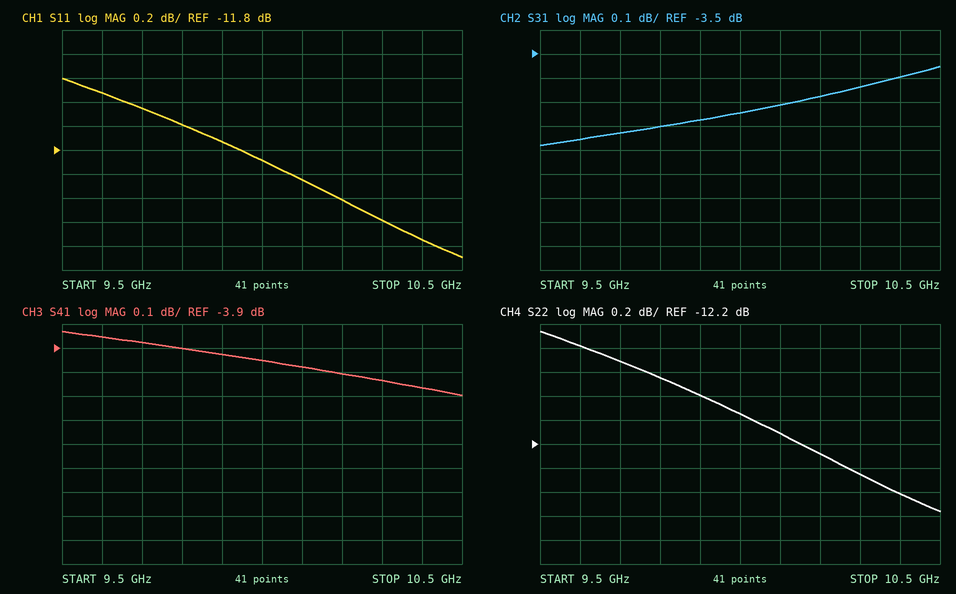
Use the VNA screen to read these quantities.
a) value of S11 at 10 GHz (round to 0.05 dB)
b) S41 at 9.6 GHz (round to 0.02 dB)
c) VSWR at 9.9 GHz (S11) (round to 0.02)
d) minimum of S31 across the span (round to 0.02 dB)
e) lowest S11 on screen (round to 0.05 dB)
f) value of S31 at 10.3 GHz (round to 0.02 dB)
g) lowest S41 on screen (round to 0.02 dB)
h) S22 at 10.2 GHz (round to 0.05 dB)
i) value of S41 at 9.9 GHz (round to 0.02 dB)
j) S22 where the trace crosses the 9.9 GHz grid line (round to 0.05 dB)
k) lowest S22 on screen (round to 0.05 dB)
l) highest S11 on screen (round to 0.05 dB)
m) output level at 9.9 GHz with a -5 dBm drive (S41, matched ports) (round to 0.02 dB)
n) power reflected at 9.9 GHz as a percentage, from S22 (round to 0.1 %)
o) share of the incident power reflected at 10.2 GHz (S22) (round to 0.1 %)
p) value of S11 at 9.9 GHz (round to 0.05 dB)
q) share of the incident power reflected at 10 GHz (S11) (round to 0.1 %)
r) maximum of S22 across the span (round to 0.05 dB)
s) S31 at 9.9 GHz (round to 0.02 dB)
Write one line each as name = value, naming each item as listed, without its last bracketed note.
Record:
value of S11 at 10 GHz = -11.90 dB
S41 at 9.6 GHz = -3.86 dB
VSWR at 9.9 GHz (S11) = 1.70
minimum of S31 across the span = -3.88 dB
lowest S11 on screen = -12.70 dB
value of S31 at 10.3 GHz = -3.64 dB
lowest S41 on screen = -4.10 dB
S22 at 10.2 GHz = -12.30 dB
value of S41 at 9.9 GHz = -3.92 dB
S22 where the trace crosses the 9.9 GHz grid line = -11.80 dB
lowest S22 on screen = -12.75 dB
highest S11 on screen = -11.20 dB
output level at 9.9 GHz with a -5 dBm drive (S41, matched ports) = -8.92 dBm
power reflected at 9.9 GHz as a percentage, from S22 = 6.6 %
share of the incident power reflected at 10.2 GHz (S22) = 5.9 %
value of S11 at 9.9 GHz = -11.75 dB
share of the incident power reflected at 10 GHz (S11) = 6.5 %
maximum of S22 across the span = -11.25 dB
S31 at 9.9 GHz = -3.78 dB
